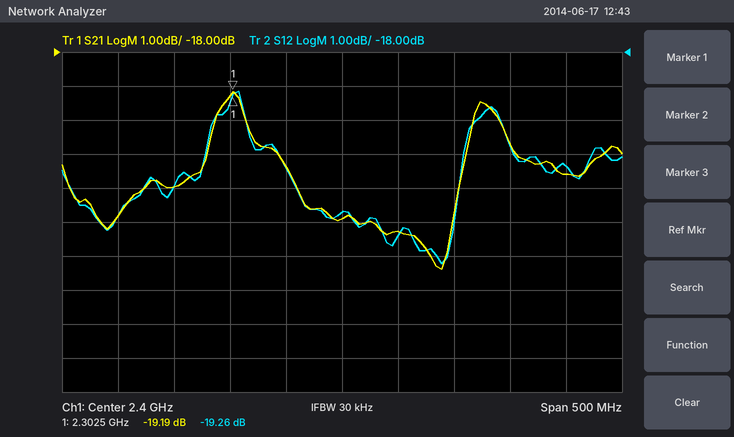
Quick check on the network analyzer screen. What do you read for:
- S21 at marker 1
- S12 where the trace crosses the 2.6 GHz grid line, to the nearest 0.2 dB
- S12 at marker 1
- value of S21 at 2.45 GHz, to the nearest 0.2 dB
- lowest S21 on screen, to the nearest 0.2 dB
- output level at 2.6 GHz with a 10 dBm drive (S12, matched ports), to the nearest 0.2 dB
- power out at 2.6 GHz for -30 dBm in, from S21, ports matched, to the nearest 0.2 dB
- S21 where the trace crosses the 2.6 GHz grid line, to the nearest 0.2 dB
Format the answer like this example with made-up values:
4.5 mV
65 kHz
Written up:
-19.19 dB
-21.4 dB
-19.26 dB
-23.2 dB
-24.4 dB
-11.4 dBm
-51.6 dBm
-21.6 dB
